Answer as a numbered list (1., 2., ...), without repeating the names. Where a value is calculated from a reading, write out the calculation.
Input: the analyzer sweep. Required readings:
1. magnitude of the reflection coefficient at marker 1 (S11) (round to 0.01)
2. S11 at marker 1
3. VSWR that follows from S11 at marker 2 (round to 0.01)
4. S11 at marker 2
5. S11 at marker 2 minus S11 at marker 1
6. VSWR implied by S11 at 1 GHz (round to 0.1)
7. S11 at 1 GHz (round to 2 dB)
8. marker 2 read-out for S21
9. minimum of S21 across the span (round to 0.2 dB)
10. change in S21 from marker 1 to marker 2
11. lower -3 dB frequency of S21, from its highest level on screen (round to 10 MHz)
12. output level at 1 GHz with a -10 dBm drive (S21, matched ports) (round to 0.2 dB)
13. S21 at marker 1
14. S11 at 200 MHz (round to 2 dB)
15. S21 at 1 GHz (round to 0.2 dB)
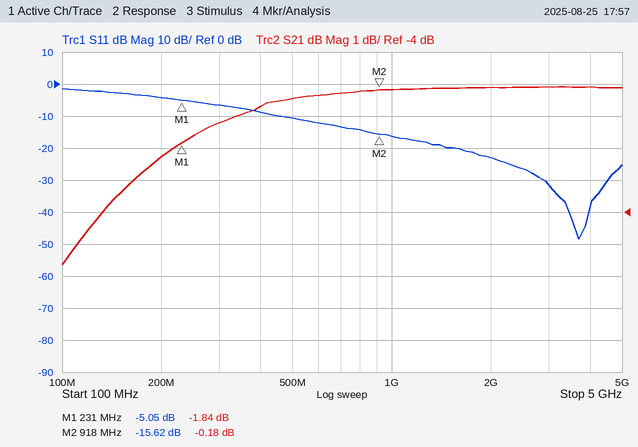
1. 10^(-5.05/20) ≈ 0.56
2. -5.05 dB
3. (1 + 0.1656)/(1 − 0.1656) ≈ 1.40
4. -15.62 dB
5. -15.62 − (-5.05) = -10.57 dB
6. |Γ| = 10^(-16/20) = 0.1585; VSWR = (1 + 0.1585)/(1 − 0.1585) ≈ 1.4
7. -16 dB
8. -0.18 dB
9. -5.6 dB
10. -0.18 − (-1.84) = 1.66 dB
11. 160 MHz
12. -10 dBm + (-0.2 dB) = -10.2 dBm
13. -1.84 dB
14. -4 dB
15. -0.2 dB
